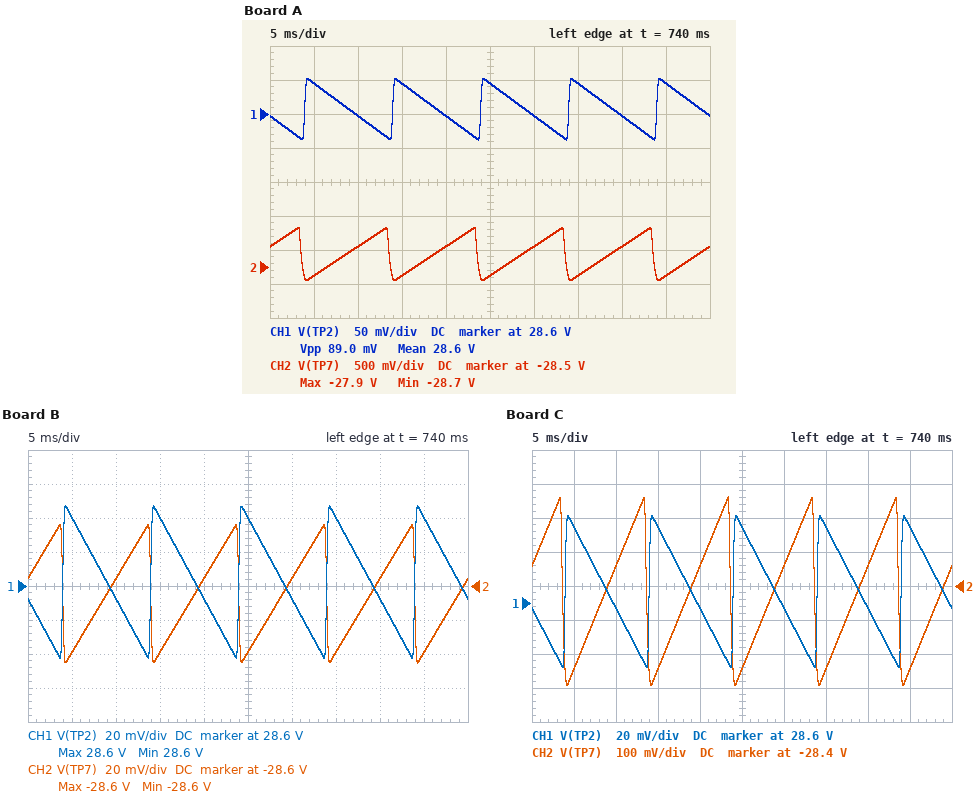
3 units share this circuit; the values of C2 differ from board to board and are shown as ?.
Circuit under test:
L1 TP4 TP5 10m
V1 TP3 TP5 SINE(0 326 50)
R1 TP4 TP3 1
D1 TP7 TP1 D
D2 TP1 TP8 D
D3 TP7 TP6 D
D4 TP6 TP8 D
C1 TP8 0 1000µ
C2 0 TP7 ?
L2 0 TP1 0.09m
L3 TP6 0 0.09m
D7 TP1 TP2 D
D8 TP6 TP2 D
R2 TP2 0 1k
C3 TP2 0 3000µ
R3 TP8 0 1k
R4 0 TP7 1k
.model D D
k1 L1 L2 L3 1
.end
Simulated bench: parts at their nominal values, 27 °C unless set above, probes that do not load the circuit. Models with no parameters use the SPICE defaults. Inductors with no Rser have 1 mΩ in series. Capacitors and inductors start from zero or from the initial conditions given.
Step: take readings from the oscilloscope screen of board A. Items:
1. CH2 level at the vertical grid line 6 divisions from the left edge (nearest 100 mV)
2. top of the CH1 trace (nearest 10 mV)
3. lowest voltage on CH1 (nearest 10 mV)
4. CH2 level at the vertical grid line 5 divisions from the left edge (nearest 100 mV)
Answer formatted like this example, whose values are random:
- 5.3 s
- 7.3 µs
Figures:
- -28.2 V
- 28.65 V
- 28.56 V
- -28.6 V
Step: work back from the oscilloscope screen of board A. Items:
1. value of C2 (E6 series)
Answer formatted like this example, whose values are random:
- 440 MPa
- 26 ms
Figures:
- 330 µF
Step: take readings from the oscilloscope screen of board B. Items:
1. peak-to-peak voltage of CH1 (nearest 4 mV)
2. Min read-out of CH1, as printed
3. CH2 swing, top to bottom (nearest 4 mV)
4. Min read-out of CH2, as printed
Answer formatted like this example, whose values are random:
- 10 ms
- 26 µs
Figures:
- 88 mV
- 28.6 V
- 80 mV
- -28.6 V
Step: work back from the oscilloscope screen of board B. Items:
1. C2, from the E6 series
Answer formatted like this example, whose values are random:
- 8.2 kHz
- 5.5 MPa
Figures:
- 3.3 mF
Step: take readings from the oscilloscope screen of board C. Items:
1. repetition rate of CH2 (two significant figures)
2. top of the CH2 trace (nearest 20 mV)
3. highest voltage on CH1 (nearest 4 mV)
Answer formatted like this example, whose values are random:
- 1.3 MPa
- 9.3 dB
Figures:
- 100 Hz
- -28.14 V
- 28.652 V
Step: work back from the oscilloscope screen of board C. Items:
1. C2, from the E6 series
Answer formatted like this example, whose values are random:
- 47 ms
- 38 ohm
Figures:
- 470 µF
